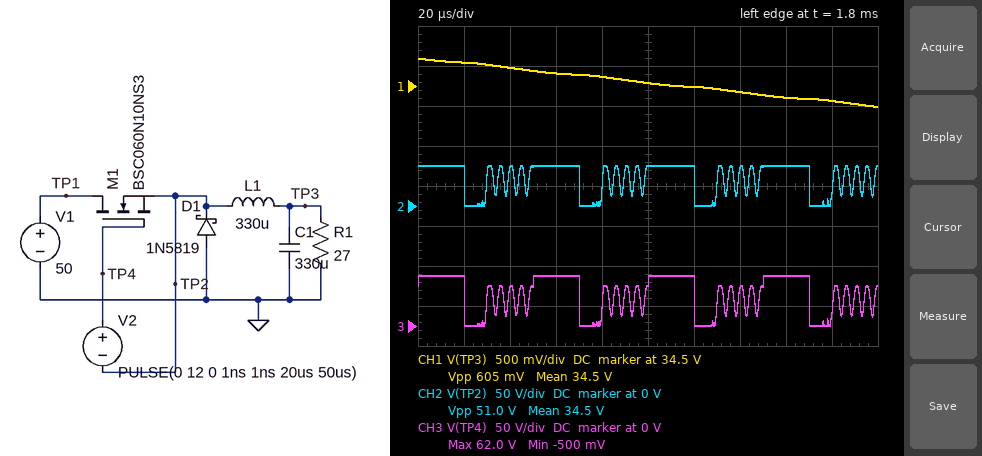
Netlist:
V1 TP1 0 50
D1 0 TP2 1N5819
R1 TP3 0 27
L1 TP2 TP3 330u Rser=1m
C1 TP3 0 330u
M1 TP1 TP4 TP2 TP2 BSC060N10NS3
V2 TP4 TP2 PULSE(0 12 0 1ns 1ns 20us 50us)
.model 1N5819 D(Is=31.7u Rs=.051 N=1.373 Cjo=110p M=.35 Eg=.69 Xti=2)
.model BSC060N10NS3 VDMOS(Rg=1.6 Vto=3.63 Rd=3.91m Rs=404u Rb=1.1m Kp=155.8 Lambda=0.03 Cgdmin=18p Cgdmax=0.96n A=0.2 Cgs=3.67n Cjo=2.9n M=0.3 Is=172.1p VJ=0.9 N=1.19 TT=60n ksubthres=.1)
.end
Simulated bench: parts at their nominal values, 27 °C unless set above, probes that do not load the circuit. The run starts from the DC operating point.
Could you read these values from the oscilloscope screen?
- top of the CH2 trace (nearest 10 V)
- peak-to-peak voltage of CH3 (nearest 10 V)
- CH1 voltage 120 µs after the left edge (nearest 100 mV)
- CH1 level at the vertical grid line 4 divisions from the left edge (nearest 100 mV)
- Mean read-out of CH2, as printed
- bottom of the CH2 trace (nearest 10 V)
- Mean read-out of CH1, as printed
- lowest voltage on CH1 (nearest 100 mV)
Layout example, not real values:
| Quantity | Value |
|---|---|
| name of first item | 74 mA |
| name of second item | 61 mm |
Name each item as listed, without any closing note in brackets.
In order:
| Quantity | Value |
|---|---|
| top of the CH2 trace | 50 V |
| peak-to-peak voltage of CH3 | 60 V |
| CH1 voltage 120 µs after the left edge | 34.5 V |
| CH1 level at the vertical grid line 4 divisions from the left edge | 34.6 V |
| Mean read-out of CH2, as printed | 34.5 V |
| bottom of the CH2 trace | 0 V |
| Mean read-out of CH1, as printed | 34.5 V |
| lowest voltage on CH1 | 34.2 V |
